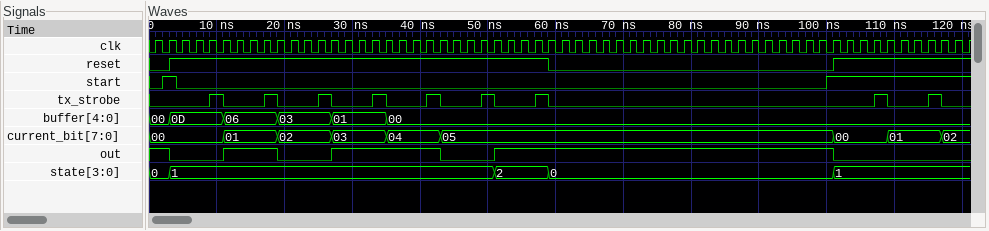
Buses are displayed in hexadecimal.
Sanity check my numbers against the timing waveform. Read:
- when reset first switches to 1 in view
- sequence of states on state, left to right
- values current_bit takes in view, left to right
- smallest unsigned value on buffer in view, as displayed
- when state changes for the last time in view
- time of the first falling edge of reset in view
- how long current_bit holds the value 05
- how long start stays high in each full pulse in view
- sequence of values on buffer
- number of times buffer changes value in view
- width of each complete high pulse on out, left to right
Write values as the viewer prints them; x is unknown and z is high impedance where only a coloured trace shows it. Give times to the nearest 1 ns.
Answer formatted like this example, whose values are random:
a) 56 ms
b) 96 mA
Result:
a) 3 ns
b) 0, 1, 2, 0, 1
c) 00, 01, 02, 03, 04, 05, 00, 01, 02
d) 00
e) 101 ns
f) 59 ns
g) 58 ns
h) 2 ns
i) 00, 0D, 06, 03, 01, 00
j) 5
k) 8 ns, 16 ns, 50 ns
